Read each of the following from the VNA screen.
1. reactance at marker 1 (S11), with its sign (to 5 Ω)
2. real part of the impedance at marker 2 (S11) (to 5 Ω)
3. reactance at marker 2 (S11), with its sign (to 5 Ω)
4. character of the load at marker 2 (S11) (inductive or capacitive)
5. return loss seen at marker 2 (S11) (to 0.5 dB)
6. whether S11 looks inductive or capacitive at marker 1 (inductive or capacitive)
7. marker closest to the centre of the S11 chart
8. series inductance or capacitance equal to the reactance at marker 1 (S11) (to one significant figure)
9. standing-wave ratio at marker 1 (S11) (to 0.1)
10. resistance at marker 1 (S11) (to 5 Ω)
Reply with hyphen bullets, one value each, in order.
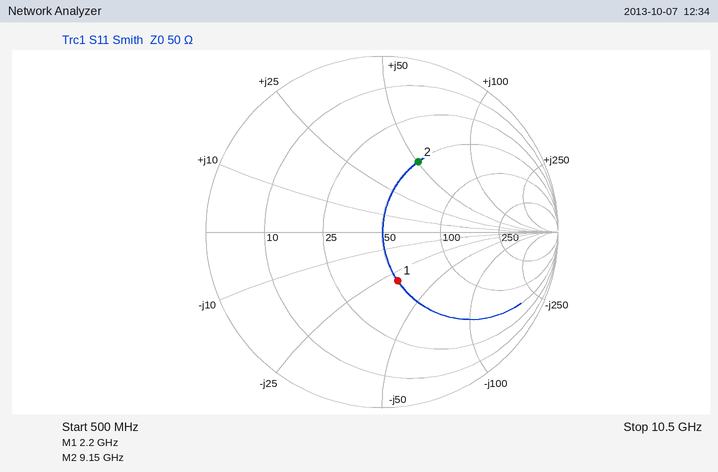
- -30 Ω
- 50 Ω
- +50 Ω
- inductive
- 7.0 dB
- capacitive
- marker 1
- 2 pF
- 1.8
- 50 Ω
